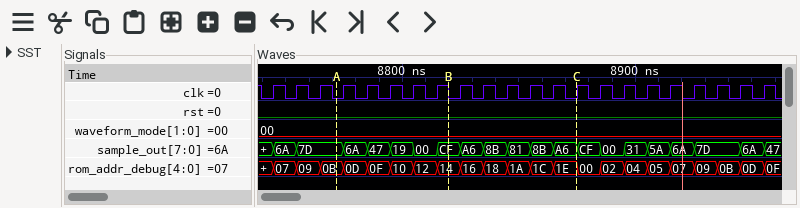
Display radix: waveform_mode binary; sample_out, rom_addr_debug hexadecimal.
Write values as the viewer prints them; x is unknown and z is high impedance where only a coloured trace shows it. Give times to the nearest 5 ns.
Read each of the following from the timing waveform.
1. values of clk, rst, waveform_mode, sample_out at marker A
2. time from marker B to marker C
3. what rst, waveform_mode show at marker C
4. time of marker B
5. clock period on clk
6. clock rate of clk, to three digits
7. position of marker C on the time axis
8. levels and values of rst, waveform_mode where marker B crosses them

clk=0, rst=0, waveform_mode=00, sample_out=7D
55 ns
rst=0, waveform_mode=00
8820 ns
10 ns
100 MHz
8875 ns
rst=0, waveform_mode=00
